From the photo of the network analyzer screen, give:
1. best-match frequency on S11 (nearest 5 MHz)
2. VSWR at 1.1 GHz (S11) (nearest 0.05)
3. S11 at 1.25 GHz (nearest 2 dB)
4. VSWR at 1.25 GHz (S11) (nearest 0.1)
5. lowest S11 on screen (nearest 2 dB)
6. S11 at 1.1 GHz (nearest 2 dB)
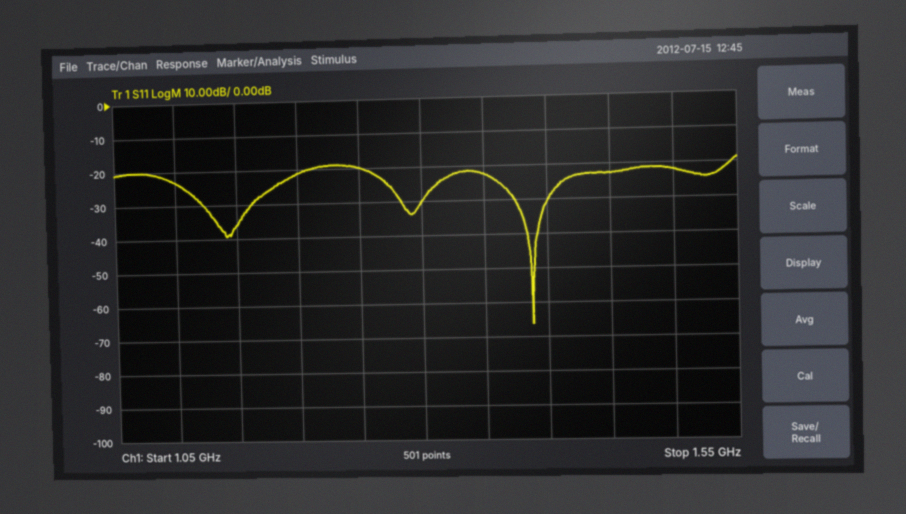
1.390 GHz
1.15
-20 dB
1.2
-66 dB
-24 dB
